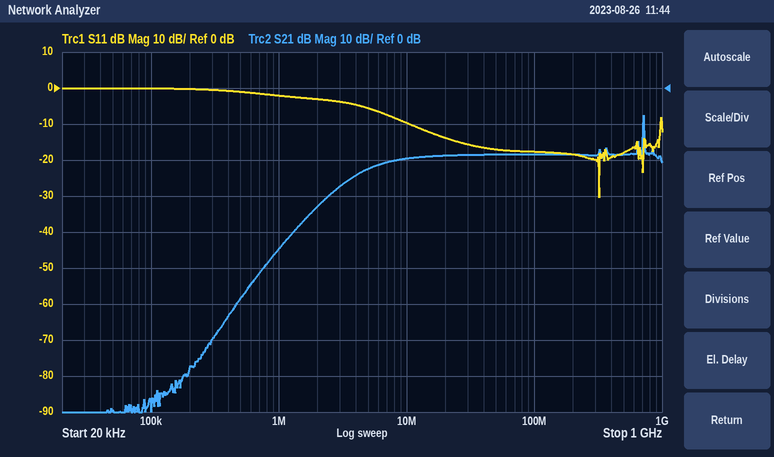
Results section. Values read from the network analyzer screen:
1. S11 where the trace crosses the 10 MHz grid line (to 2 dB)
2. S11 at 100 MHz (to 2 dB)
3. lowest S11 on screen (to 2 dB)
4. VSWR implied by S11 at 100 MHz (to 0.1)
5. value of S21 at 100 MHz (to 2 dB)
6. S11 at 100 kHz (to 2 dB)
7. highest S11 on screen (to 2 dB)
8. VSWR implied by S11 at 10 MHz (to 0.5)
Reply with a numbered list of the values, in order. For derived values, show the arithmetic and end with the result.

1. -10 dB
2. -18 dB
3. -30 dB
4. |Γ| = 10^(-18/20) = 0.1259; VSWR = (1 + 0.1259)/(1 − 0.1259) ≈ 1.3
5. -18 dB
6. 0 dB
7. 0 dB
8. |Γ| = 10^(-10/20) = 0.3162; VSWR = (1 + 0.3162)/(1 − 0.3162) ≈ 1.92, so 2.0 to the nearest 0.5
